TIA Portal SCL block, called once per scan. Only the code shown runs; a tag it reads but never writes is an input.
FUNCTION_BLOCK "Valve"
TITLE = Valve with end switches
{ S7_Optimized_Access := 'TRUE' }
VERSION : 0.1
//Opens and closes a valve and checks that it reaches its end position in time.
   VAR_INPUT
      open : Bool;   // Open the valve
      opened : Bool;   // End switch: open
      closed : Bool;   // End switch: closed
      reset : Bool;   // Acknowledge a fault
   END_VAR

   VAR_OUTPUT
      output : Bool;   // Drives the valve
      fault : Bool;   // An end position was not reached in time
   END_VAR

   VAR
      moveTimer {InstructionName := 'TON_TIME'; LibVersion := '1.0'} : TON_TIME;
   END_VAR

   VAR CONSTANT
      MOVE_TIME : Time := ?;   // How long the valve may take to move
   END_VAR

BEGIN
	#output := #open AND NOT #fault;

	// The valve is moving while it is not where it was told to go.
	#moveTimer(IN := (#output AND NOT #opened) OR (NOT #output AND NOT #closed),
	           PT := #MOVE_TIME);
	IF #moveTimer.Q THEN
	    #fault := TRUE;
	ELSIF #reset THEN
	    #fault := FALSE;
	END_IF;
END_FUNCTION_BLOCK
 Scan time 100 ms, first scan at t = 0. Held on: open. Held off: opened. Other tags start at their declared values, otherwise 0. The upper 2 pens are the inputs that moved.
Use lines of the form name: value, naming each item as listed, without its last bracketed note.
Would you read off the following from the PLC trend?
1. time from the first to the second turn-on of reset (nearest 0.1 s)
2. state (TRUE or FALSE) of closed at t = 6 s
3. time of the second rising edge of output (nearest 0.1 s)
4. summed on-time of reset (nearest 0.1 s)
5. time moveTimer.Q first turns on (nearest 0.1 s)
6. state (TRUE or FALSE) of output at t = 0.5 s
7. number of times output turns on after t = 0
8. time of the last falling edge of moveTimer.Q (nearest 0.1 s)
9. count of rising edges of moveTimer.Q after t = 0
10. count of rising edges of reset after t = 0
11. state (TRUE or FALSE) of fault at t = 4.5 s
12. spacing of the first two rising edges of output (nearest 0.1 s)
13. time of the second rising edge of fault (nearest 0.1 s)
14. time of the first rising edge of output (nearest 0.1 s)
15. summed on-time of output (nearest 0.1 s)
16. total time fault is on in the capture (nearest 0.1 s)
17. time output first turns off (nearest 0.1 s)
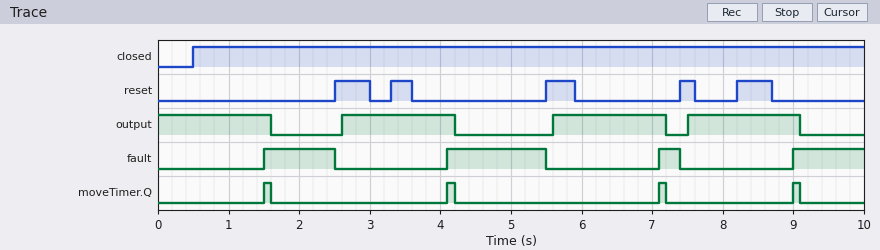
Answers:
time from the first to the second turn-on of reset: 0.8 s
state (TRUE or FALSE) of closed at t = 6 s: TRUE
time of the second rising edge of output: 5.6 s
summed on-time of reset: 1.9 s
time moveTimer.Q first turns on: 1.5 s
state (TRUE or FALSE) of output at t = 0.5 s: TRUE
number of times output turns on after t = 0: 3
time of the last falling edge of moveTimer.Q: 9.1 s
count of rising edges of moveTimer.Q after t = 0: 4
count of rising edges of reset after t = 0: 5
state (TRUE or FALSE) of fault at t = 4.5 s: TRUE
spacing of the first two rising edges of output: 3.0 s
time of the second rising edge of fault: 4.1 s
time of the first rising edge of output: 2.6 s
summed on-time of output: 6.4 s
total time fault is on in the capture: 3.7 s
time output first turns off: 1.6 s
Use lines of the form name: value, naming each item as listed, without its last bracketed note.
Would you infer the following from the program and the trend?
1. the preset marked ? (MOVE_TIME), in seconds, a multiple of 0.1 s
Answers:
the preset marked ? (MOVE_TIME), in seconds, a multiple of 0.1 s: 1.5 s
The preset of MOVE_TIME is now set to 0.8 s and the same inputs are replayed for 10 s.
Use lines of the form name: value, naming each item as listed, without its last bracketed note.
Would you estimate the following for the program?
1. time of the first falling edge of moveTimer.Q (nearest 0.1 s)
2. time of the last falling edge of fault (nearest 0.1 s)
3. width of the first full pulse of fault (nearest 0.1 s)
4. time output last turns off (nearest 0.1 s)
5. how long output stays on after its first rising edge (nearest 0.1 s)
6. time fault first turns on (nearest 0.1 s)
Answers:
time of the first falling edge of moveTimer.Q: 0.9 s
time of the last falling edge of fault: 8.4 s
width of the first full pulse of fault: 1.7 s
time output last turns off: 9.4 s
how long output stays on after its first rising edge: 0.9 s
time fault first turns on: 0.8 s
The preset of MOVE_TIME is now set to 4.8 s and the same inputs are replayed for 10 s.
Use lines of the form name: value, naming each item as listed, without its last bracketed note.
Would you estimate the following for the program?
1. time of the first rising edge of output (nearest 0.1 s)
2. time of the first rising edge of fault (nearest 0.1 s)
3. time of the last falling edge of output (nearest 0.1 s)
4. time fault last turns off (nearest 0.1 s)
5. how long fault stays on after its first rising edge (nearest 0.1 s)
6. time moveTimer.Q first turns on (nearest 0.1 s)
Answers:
time of the first rising edge of output: 5.6 s
time of the first rising edge of fault: 4.8 s
time of the last falling edge of output: 4.9 s
time fault last turns off: 5.5 s
how long fault stays on after its first rising edge: 0.7 s
time moveTimer.Q first turns on: 4.8 s
